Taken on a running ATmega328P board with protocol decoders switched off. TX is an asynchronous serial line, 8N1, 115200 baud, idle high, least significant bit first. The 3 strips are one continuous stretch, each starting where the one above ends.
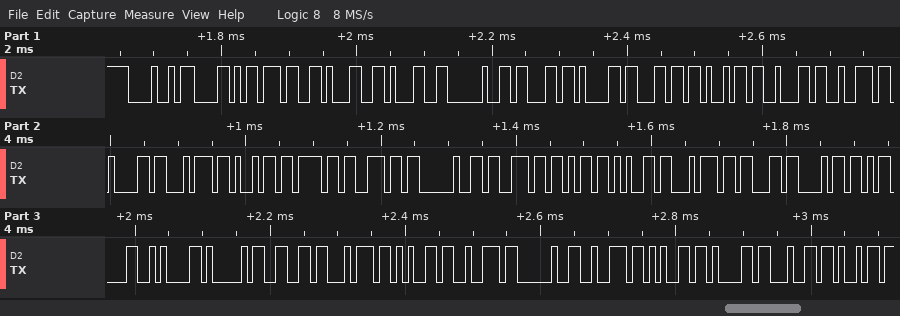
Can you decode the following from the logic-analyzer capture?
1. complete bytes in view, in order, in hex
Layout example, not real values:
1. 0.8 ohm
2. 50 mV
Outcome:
1. 0x48 0x58 0x37 0x31 0x31 0x20 0x63 0x61 0x6C 0x69 0x62 0x72 0x61 0x74 0x69 0x6F 0x6E 0x20 0x73 0x6B 0x65 0x74 0x63 0x68 0x0D 0x0A 0x41 0x66 0x74 0x65 0x72 0x20 0x72 0x65 0x61 0x64 0x69
